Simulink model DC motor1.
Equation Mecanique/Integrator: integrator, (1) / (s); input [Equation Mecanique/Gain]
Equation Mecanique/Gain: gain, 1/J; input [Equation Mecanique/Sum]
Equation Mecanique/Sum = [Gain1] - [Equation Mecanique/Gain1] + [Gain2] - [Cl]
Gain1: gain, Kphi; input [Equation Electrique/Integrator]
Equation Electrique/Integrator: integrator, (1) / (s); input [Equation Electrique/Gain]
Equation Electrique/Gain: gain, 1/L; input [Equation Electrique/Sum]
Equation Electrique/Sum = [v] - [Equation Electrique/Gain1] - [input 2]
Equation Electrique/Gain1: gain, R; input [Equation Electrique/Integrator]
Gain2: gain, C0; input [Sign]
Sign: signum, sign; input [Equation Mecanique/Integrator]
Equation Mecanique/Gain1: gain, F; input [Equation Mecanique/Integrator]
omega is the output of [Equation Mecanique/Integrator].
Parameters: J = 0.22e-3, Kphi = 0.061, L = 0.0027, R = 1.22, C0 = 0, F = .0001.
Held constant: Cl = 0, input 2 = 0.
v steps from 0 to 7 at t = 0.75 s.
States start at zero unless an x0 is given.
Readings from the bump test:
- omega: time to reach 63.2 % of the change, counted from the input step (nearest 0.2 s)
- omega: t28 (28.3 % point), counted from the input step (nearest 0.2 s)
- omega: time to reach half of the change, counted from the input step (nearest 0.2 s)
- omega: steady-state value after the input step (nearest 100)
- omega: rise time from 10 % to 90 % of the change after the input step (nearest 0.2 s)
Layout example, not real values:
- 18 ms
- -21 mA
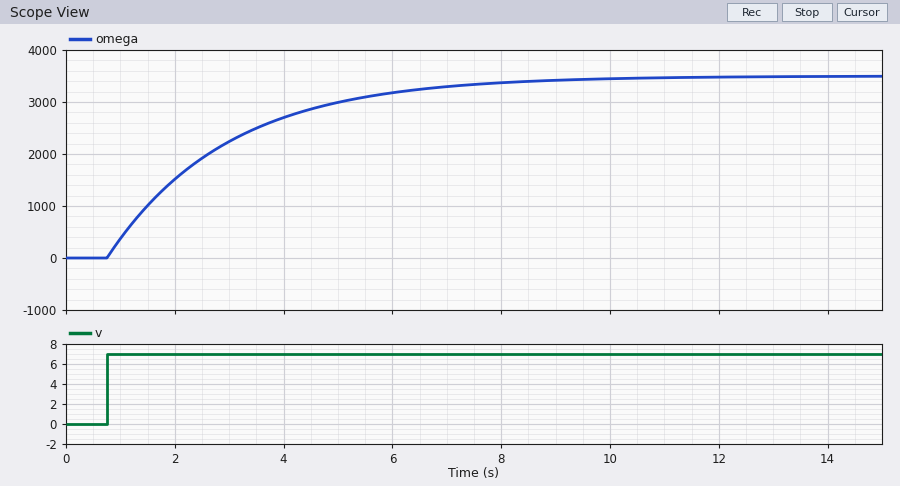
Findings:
- 2.2 s
- 0.8 s
- 1.6 s
- 3500
- 4.8 s
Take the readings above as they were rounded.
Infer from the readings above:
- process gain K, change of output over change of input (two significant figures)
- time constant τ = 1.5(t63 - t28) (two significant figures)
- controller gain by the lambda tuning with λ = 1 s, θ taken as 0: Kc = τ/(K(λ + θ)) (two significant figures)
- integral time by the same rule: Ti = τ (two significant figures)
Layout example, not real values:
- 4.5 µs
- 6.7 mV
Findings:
- 500
- 2.1 s
- 0.0042
- 2.1 s
